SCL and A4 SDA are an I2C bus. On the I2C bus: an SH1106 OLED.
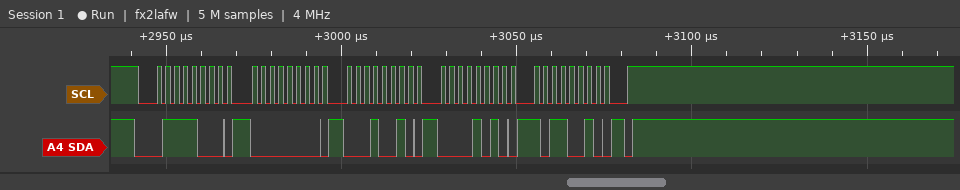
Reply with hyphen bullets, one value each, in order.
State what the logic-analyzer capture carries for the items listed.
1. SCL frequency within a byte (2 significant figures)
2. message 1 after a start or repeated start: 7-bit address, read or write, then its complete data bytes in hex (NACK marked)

- 400 kHz
- 0x3C write: 00 12 0A B2
